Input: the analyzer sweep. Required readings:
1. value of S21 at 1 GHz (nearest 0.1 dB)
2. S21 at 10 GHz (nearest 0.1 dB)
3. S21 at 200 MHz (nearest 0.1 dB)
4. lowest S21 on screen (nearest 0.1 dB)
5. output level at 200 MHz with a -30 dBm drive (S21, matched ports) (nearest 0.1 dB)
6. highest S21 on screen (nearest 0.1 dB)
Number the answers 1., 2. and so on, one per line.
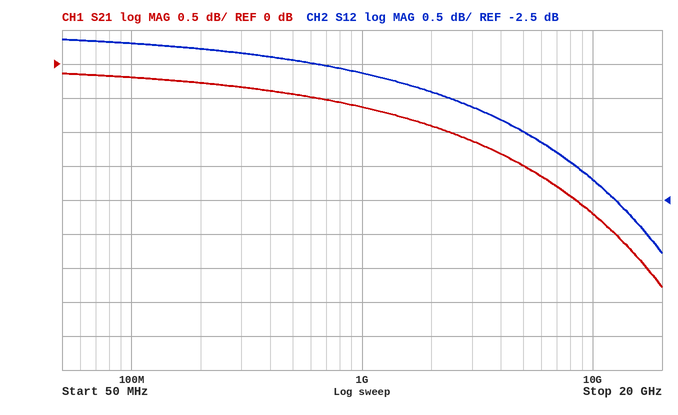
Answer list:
1. -0.6 dB
2. -2.2 dB
3. -0.3 dB
4. -3.3 dB
5. -30.3 dBm
6. -0.1 dB
